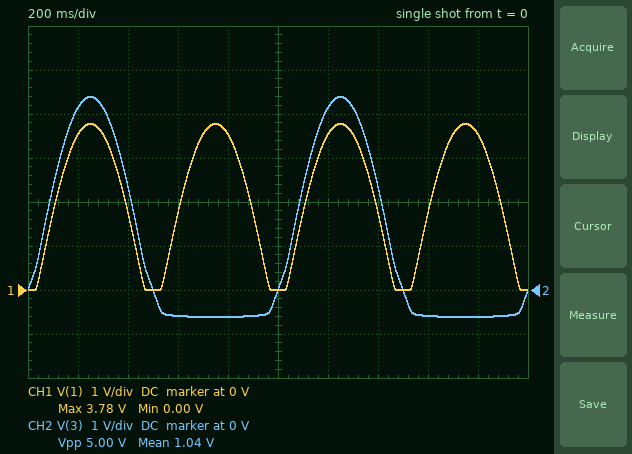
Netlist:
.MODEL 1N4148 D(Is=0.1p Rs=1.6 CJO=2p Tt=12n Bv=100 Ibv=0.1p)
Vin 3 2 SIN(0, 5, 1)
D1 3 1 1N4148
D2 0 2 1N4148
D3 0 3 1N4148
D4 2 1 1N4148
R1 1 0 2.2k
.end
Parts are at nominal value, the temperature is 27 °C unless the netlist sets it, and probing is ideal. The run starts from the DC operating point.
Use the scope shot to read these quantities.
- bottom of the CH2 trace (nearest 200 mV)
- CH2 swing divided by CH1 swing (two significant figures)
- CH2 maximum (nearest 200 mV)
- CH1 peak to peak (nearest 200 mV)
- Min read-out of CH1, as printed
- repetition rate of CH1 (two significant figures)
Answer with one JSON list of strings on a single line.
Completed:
["-600 mV", "1.3", "4.4 V", "3.8 V", "0.00 V", "2.0 Hz"]
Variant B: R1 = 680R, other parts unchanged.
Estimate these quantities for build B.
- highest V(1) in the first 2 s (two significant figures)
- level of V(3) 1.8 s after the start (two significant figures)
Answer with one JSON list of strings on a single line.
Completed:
["3.7 V", "-650 mV"]
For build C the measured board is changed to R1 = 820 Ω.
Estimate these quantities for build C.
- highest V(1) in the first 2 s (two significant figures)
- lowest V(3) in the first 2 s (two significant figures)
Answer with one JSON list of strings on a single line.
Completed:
["3.7 V", "-640 mV"]
